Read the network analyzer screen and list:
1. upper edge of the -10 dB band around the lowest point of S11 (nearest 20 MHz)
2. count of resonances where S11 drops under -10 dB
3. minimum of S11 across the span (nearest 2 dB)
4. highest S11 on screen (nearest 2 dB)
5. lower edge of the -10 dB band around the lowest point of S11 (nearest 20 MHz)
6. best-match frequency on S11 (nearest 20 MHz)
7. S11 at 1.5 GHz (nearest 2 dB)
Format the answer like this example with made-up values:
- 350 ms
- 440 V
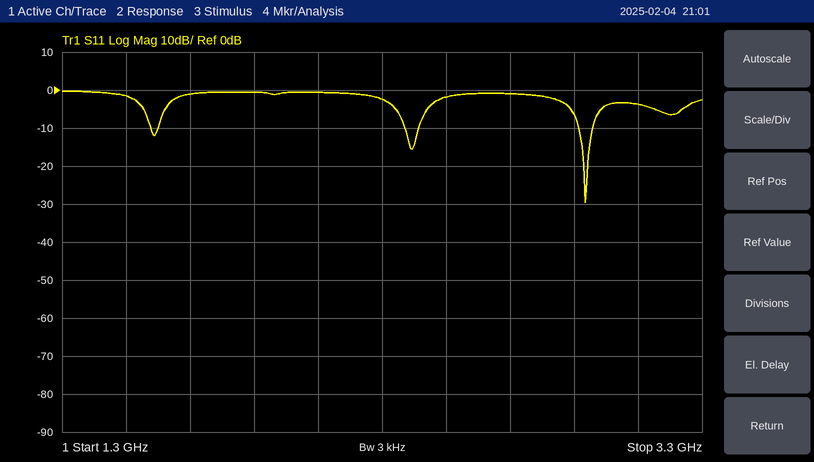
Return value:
- 2.96 GHz
- 3
- -30 dB
- 0 dB
- 2.92 GHz
- 2.94 GHz
- -2 dB
